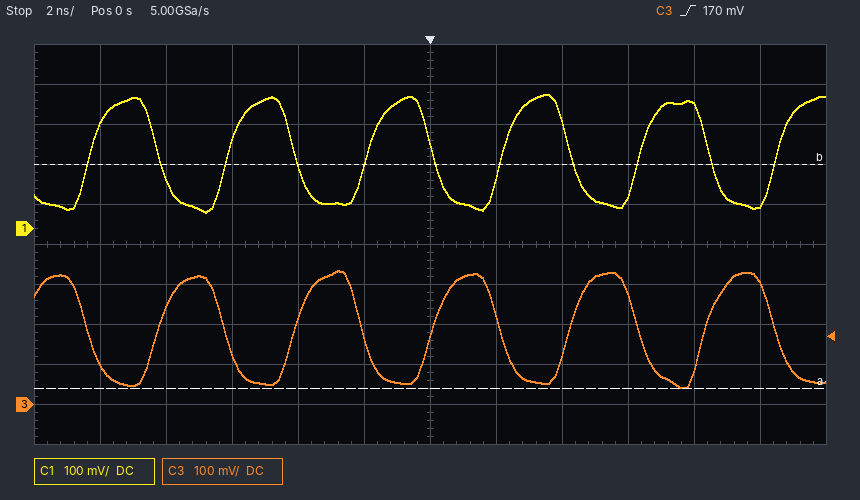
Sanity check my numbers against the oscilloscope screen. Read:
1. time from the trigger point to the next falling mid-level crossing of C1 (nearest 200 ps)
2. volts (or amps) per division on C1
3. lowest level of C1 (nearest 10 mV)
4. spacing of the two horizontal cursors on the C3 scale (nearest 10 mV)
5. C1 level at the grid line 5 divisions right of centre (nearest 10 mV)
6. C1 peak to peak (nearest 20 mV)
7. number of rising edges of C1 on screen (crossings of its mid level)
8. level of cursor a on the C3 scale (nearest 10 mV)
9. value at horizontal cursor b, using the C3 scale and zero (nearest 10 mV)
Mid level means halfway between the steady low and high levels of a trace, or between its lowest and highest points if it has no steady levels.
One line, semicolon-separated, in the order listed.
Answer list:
4.2 ns; 100 mV; 40 mV; 560 mV; 60 mV; 300 mV; 6; 40 mV; 600 mV
